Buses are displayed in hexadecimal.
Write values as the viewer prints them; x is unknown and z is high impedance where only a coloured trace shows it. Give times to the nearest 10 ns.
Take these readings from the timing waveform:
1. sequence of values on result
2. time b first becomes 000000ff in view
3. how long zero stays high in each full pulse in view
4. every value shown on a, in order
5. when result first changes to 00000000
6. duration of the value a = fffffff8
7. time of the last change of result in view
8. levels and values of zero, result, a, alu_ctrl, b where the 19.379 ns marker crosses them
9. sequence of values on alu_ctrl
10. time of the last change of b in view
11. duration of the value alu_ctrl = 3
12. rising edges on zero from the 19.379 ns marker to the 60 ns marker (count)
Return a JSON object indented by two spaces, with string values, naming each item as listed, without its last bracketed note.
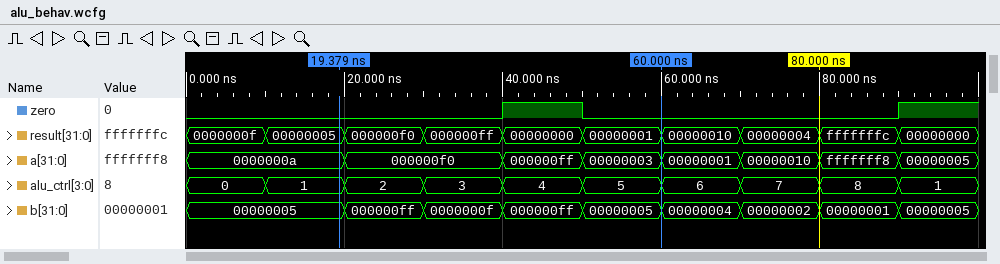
{
  "sequence of values on result": "0000000f, 00000005, 000000f0, 000000ff, 00000000, 00000001, 00000010, 00000004, fffffffc, 00000000",
  "time b first becomes 000000ff in view": "20 ns",
  "how long zero stays high in each full pulse in view": "10 ns",
  "every value shown on a, in order": "0000000a, 000000f0, 000000ff, 00000003, 00000001, 00000010, fffffff8, 00000005",
  "when result first changes to 00000000": "40 ns",
  "duration of the value a = fffffff8": "10 ns",
  "time of the last change of result in view": "90 ns",
  "levels and values of zero, result, a, alu_ctrl, b where the 19.379 ns marker crosses them": "zero=0, result=00000005, a=0000000a, alu_ctrl=1, b=00000005",
  "sequence of values on alu_ctrl": "0, 1, 2, 3, 4, 5, 6, 7, 8, 1",
  "time of the last change of b in view": "90 ns",
  "duration of the value alu_ctrl = 3": "10 ns",
  "rising edges on zero from the 19.379 ns marker to the 60 ns marker": "1"
}
